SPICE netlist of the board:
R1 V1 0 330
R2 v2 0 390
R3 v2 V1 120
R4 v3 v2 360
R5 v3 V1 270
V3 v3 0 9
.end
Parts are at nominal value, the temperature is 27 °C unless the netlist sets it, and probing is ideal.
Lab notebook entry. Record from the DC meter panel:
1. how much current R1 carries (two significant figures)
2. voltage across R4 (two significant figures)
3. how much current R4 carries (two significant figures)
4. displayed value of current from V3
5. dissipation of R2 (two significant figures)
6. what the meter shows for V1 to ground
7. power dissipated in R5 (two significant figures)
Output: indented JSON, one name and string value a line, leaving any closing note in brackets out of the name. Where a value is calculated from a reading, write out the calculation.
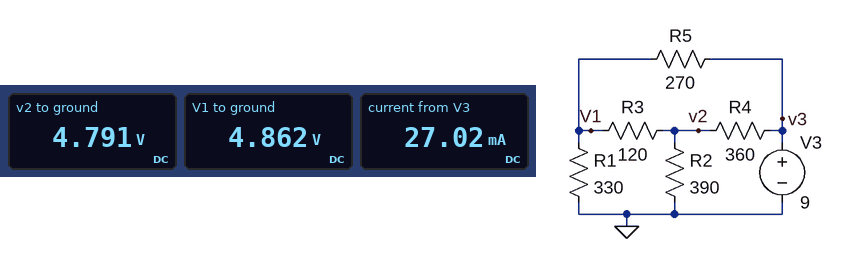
{
  "how much current R1 carries": "(4.862 V) / 330 Ω = 15 mA",
  "voltage across R4": "9 V - 4.791 V = 4.2 V",
  "how much current R4 carries": "(9 V - 4.791 V) / 360 Ω = 12 mA",
  "displayed value of current from V3": "27.02 mA",
  "dissipation of R2": "(4.791 V)^2 / 390 Ω = 59 mW",
  "what the meter shows for V1 to ground": "4.862 V",
  "power dissipated in R5": "(9 V - 4.862 V)^2 / 270 Ω = 63 mW"
}
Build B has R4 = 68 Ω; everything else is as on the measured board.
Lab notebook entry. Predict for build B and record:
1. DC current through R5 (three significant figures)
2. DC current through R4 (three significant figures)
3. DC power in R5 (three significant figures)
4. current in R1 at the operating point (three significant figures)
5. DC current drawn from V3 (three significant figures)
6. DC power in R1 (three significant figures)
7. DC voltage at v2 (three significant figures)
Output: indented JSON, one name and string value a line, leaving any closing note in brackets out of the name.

{
  "DC current through R5": "10.4 mA",
  "DC current through R4": "26.7 mA",
  "DC power in R5": "29.4 mW",
  "current in R1 at the operating point": "18.7 mA",
  "DC current drawn from V3": "37.2 mA",
  "DC power in R1": "116 mW",
  "DC voltage at v2": "7.18 V"
}
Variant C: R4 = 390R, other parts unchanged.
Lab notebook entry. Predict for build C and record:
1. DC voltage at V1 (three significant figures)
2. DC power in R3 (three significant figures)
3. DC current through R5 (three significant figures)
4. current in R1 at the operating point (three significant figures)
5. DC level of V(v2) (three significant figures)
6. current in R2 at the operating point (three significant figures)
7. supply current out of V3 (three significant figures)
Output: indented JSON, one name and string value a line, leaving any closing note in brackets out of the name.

{
  "DC voltage at V1": "4.81 V",
  "DC power in R3": "113 µW",
  "DC current through R5": "15.5 mA",
  "current in R1 at the operating point": "14.6 mA",
  "DC level of V(v2)": "4.69 V",
  "current in R2 at the operating point": "12.0 mA",
  "supply current out of V3": "26.6 mA"
}
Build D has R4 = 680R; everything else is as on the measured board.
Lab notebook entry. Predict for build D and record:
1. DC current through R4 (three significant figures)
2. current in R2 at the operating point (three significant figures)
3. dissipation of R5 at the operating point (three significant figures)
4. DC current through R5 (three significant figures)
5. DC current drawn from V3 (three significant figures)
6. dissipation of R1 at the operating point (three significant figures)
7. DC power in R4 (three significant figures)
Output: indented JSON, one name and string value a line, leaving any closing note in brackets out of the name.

{
  "DC current through R4": "7.23 mA",
  "current in R2 at the operating point": "10.5 mA",
  "dissipation of R5 at the operating point": "76.0 mW",
  "DC current through R5": "16.8 mA",
  "DC current drawn from V3": "24.0 mA",
  "dissipation of R1 at the operating point": "60.5 mW",
  "DC power in R4": "35.6 mW"
}
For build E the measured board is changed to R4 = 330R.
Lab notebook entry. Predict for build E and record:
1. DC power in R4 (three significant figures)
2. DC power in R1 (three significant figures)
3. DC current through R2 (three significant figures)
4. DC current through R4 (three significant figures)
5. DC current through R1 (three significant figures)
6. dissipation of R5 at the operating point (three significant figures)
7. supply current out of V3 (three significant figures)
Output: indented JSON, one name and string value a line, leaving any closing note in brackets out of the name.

{
  "DC power in R4": "50.8 mW",
  "DC power in R1": "73.5 mW",
  "DC current through R2": "12.6 mA",
  "DC current through R4": "12.4 mA",
  "DC current through R1": "14.9 mA",
  "dissipation of R5 at the operating point": "61.5 mW",
  "supply current out of V3": "27.5 mA"
}
